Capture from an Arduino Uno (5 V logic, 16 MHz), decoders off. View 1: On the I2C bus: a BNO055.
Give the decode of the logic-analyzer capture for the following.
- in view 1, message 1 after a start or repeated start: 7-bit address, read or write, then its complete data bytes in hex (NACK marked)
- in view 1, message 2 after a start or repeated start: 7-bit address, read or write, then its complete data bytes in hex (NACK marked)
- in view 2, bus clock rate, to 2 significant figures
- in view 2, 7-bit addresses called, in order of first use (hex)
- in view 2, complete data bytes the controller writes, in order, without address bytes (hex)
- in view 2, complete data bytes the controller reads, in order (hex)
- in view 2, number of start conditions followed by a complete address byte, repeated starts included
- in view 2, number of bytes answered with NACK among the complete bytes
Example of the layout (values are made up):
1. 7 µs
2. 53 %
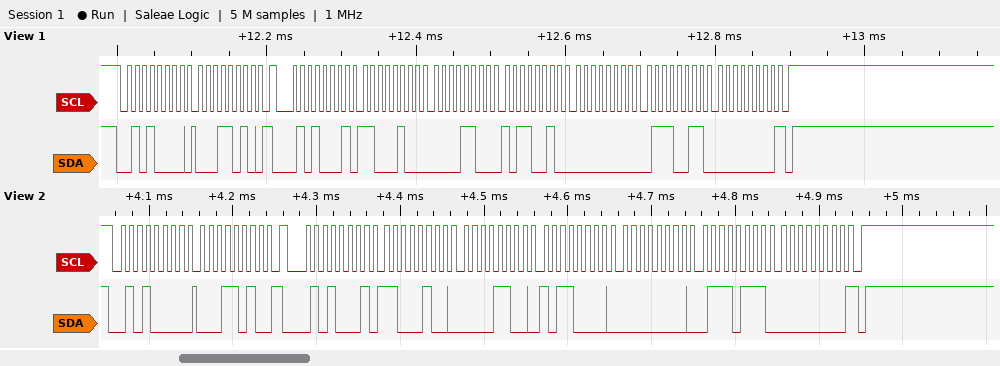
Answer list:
1. 0x28 write: 1A
2. 0x28 read: C4 0C B2 00 73 00 NACK
3. 100 kHz
4. 0x28
5. 1A
6. C4 0C B0 00 77 00
7. 2
8. 1
